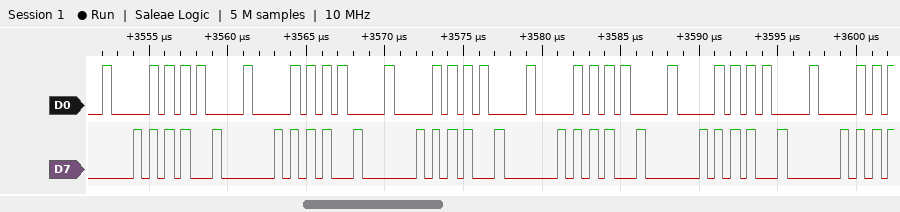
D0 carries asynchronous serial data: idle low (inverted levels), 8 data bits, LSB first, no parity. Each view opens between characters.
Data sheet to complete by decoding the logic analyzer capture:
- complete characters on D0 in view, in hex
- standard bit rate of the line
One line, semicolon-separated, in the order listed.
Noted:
5F, 7D, D5, 5F, 7D, D5, 5F, 7D; 2000000 baud
